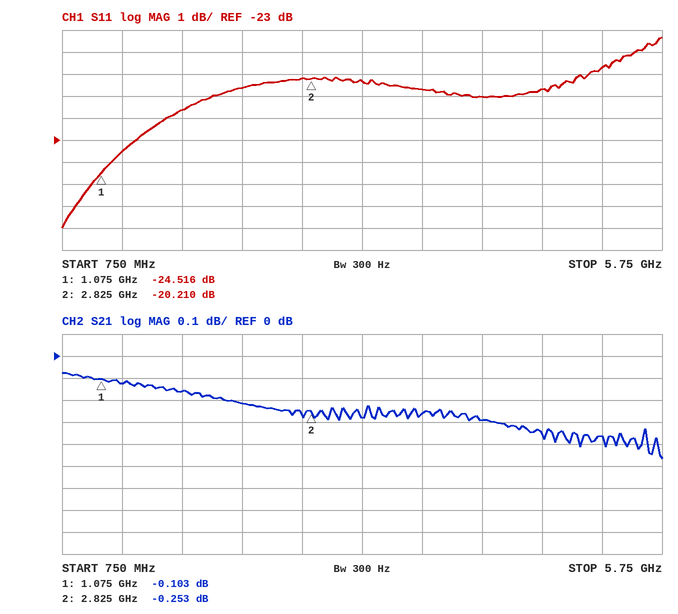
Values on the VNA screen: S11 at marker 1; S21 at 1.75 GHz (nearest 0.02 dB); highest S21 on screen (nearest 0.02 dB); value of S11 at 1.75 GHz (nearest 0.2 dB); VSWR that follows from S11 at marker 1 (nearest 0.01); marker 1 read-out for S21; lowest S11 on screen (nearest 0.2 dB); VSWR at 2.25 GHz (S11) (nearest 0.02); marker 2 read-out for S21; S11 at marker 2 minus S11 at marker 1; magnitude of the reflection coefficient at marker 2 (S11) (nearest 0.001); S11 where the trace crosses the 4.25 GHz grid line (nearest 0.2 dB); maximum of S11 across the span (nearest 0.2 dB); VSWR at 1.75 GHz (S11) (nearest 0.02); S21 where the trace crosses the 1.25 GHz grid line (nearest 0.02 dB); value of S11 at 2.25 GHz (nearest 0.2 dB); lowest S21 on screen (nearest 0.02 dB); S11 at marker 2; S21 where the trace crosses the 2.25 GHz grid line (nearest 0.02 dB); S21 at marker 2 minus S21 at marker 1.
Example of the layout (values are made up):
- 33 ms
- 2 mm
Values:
- -24.516 dB
- -0.16 dB
- -0.08 dB
- -21.6 dB
- 1.13
- -0.103 dB
- -27.0 dB
- 1.20
- -0.253 dB
- 4.306 dB
- 0.098
- -21.0 dB
- -18.4 dB
- 1.18
- -0.12 dB
- -20.6 dB
- -0.46 dB
- -20.210 dB
- -0.22 dB
- -0.150 dB
